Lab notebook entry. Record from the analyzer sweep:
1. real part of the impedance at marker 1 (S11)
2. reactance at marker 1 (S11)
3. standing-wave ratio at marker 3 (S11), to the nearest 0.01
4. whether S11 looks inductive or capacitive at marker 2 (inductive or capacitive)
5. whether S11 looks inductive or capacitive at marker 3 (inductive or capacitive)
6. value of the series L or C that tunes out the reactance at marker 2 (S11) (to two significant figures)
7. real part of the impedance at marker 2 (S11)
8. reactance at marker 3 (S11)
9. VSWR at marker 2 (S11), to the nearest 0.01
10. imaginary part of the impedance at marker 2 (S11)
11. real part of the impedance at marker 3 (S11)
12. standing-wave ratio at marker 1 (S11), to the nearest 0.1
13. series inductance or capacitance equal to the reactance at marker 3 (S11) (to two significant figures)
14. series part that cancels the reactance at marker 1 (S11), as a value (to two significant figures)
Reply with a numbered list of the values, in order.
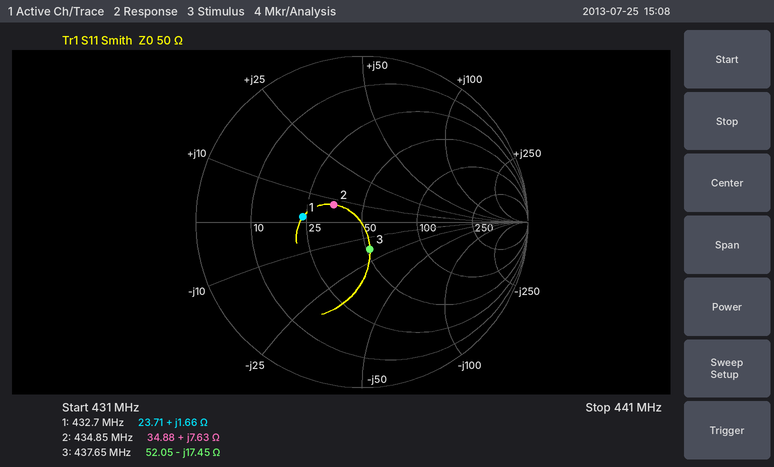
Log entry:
1. 23.71 Ω
2. +1.66 Ω
3. 1.41
4. inductive
5. capacitive
6. 48 pF
7. 34.88 Ω
8. -17.45 Ω
9. 1.50
10. +7.63 Ω
11. 52.05 Ω
12. 2.1
13. 21 pF
14. 220 pF
